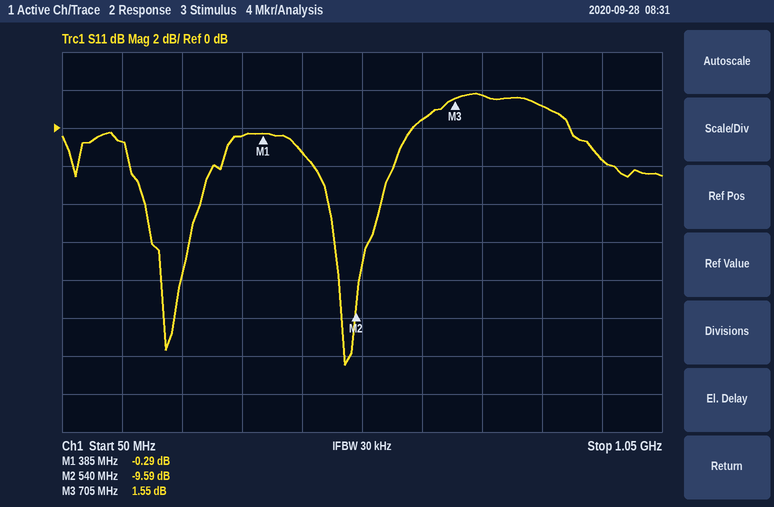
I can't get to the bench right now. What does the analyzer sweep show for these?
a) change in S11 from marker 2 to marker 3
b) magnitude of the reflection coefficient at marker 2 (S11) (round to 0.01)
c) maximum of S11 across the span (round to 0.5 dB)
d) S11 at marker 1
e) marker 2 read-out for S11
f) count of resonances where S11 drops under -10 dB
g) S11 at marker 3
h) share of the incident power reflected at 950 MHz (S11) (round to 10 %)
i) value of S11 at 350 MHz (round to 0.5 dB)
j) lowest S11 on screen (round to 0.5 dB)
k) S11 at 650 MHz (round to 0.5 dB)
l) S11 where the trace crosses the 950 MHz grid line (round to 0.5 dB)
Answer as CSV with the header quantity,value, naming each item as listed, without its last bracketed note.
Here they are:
quantity,value
change in S11 from marker 2 to marker 3,11.14 dB
magnitude of the reflection coefficient at marker 2 (S11),0.33
maximum of S11 across the span,2.0 dB
S11 at marker 1,-0.29 dB
marker 2 read-out for S11,-9.59 dB
count of resonances where S11 drops under -10 dB,2
S11 at marker 3,1.55 dB
share of the incident power reflected at 950 MHz (S11),70 %
value of S11 at 350 MHz,-0.5 dB
lowest S11 on screen,-12.5 dB
S11 at 650 MHz,0.5 dB
S11 where the trace crosses the 950 MHz grid line,-1.5 dB
